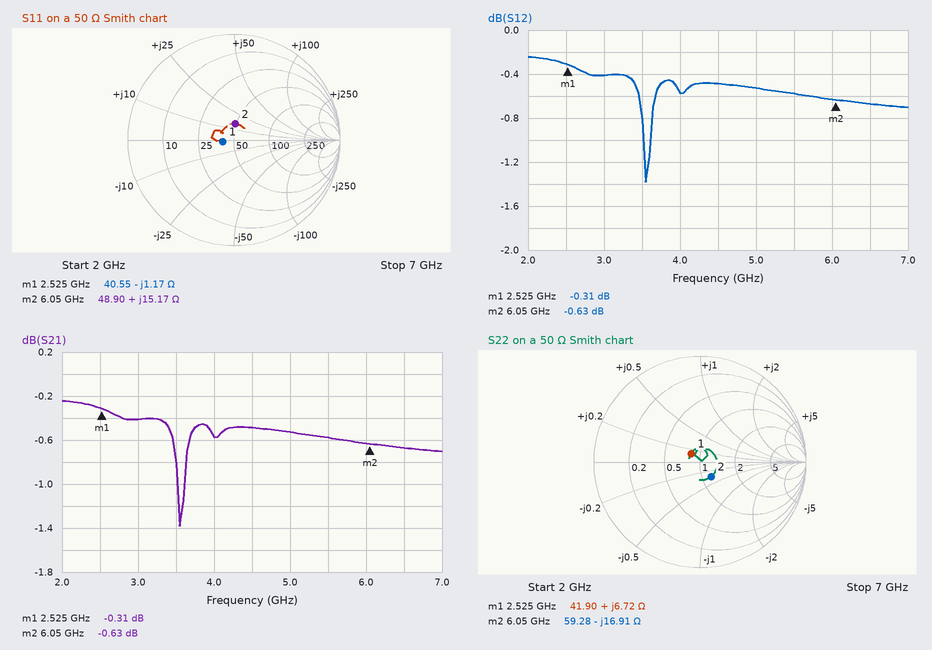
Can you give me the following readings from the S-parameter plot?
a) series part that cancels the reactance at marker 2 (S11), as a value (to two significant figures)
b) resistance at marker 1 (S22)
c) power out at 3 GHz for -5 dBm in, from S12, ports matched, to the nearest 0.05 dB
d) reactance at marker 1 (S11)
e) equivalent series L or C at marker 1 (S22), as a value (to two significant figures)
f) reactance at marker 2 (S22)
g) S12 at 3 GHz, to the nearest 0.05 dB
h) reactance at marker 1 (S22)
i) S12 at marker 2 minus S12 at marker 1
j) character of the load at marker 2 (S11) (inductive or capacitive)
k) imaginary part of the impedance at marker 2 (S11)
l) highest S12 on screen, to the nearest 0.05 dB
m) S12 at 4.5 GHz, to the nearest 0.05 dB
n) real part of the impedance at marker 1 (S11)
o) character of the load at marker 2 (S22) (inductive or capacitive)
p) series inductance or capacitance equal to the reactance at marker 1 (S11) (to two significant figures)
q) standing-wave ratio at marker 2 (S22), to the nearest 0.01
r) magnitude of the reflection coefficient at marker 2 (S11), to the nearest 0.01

1.7 pF
41.90 Ω
-5.40 dBm
-1.17 Ω
420 pH
-16.91 Ω
-0.40 dB
+6.72 Ω
-0.32 dB
inductive
+15.17 Ω
-0.25 dB
-0.50 dB
40.55 Ω
capacitive
54 pF
1.42
0.15
